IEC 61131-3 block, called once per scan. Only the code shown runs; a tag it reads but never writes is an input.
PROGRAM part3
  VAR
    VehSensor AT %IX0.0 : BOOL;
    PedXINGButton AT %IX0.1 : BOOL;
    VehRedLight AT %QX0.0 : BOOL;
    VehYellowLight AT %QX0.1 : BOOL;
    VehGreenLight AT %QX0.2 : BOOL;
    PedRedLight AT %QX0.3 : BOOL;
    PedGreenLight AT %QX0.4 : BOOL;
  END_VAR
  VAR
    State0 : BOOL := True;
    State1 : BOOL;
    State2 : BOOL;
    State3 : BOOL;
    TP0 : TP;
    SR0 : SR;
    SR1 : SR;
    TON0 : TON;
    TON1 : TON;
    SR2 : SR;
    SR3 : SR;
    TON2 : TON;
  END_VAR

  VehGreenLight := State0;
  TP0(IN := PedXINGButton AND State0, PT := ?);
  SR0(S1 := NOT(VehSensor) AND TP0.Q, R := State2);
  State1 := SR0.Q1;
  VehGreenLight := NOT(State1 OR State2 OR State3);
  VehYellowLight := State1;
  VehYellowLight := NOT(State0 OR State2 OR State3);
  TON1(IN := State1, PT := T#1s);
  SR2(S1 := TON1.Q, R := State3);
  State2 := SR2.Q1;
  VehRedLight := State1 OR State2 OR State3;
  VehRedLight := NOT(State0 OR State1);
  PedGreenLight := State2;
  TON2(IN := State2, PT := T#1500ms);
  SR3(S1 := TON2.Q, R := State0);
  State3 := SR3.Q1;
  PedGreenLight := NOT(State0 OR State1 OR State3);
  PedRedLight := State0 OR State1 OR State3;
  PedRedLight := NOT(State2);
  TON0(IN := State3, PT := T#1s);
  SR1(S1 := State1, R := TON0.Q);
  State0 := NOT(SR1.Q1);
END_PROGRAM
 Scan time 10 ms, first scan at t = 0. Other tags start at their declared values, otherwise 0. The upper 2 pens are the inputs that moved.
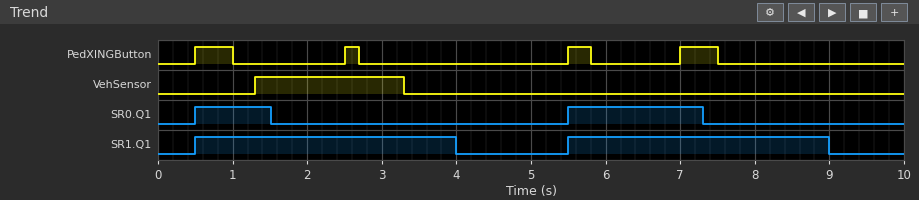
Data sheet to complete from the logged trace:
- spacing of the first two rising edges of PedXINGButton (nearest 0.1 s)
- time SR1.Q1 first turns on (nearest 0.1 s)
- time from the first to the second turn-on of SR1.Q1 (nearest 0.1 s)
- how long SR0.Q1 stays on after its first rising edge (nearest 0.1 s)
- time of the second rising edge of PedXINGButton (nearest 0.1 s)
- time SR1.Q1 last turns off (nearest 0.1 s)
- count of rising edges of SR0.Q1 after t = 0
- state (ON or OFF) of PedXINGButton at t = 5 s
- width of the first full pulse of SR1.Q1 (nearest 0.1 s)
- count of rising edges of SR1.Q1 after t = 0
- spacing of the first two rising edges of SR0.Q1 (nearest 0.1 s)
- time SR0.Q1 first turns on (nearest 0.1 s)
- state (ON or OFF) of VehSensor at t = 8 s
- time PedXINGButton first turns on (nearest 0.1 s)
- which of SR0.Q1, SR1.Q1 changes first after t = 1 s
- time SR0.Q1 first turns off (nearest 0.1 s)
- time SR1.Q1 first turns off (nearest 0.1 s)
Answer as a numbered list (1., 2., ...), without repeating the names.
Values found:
1. 2.0 s
2. 0.5 s
3. 5.0 s
4. 1.0 s
5. 2.5 s
6. 9.0 s
7. 2
8. OFF
9. 3.5 s
10. 2
11. 5.0 s
12. 0.5 s
13. OFF
14. 0.5 s
15. SR0.Q1
16. 1.5 s
17. 4.0 s
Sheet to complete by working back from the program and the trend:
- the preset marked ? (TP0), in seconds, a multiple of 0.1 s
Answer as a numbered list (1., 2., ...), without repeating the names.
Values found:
1. 1.8 s
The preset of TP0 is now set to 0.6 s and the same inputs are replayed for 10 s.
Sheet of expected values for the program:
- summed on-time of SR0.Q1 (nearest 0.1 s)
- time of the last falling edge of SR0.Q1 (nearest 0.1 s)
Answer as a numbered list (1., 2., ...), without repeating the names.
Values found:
1. 2.0 s
2. 6.5 s
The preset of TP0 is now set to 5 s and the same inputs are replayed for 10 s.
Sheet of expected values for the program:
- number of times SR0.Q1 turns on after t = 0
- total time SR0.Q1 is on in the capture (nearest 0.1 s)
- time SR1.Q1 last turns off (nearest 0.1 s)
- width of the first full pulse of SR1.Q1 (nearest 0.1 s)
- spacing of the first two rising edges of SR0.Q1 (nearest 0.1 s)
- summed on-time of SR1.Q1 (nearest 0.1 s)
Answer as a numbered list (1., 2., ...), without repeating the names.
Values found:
1. 3
2. 7.7 s
3. 5.5 s
4. 5.0 s
5. 2.8 s
6. 9.5 s
